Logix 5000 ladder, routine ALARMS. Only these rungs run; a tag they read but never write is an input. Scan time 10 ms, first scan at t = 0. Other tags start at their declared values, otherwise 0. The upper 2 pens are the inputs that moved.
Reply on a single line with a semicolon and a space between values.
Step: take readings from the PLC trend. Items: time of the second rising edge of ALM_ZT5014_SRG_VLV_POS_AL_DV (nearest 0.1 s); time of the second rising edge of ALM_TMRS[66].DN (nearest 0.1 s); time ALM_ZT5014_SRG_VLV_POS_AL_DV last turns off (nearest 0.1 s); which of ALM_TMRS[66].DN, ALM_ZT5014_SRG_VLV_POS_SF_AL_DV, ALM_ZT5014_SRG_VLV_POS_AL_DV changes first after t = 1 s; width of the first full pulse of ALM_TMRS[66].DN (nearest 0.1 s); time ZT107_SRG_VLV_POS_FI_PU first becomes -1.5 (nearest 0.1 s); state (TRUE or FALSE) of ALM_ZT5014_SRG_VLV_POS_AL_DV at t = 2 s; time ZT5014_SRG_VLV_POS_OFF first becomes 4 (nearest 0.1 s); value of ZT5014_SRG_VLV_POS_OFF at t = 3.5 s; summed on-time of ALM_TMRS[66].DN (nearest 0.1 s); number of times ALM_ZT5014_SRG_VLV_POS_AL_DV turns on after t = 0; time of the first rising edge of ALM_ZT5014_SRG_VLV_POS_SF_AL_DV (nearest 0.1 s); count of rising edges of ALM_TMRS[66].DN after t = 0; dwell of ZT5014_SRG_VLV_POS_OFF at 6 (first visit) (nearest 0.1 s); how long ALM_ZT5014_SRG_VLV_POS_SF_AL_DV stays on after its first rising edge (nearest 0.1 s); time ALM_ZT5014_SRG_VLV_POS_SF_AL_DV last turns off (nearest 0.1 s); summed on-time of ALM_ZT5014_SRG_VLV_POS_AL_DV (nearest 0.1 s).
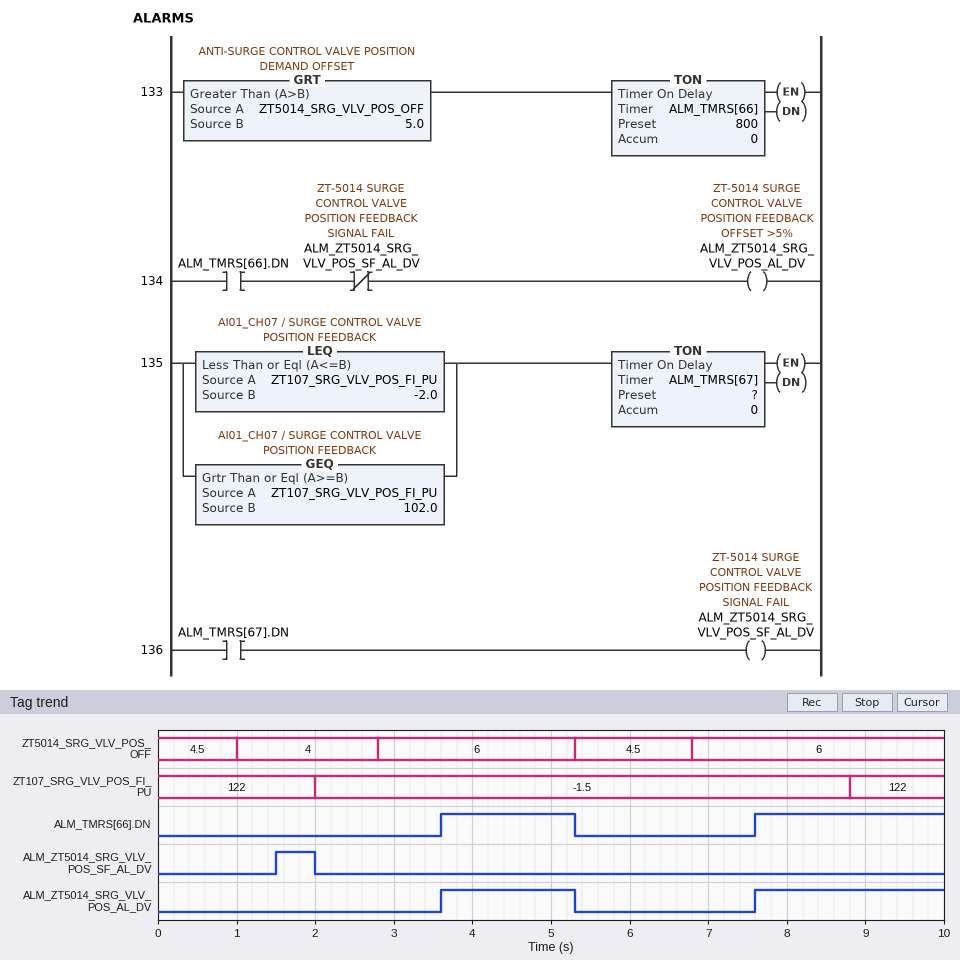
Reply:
7.6 s; 7.6 s; 5.3 s; ALM_ZT5014_SRG_VLV_POS_SF_AL_DV; 1.7 s; 2.0 s; FALSE; 1.0 s; 6; 4.1 s; 2; 1.5 s; 2; 2.5 s; 0.5 s; 2.0 s; 4.1 s
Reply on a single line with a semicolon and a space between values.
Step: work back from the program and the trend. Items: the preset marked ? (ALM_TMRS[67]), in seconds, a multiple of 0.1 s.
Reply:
1.5 s
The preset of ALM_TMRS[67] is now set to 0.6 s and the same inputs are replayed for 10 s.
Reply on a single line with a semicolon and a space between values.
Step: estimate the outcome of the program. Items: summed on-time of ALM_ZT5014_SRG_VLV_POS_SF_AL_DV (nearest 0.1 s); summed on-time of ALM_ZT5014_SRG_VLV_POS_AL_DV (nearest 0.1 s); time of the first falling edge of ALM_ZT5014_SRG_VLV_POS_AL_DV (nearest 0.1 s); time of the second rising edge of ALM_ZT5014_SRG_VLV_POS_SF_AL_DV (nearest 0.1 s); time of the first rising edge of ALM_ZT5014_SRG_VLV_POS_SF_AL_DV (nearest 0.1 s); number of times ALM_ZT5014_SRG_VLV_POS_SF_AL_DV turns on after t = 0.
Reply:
2.0 s; 3.5 s; 5.3 s; 9.4 s; 0.6 s; 2
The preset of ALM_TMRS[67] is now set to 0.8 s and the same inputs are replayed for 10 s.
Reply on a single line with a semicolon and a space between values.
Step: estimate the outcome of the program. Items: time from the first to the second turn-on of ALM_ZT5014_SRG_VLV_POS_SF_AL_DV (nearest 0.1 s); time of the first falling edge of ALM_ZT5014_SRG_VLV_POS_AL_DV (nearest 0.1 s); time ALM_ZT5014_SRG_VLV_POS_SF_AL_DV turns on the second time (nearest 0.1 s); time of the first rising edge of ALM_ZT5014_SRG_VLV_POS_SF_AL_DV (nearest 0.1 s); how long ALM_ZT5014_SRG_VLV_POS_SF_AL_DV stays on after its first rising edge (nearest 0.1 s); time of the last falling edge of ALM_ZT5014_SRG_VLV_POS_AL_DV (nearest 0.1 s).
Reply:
8.8 s; 5.3 s; 9.6 s; 0.8 s; 1.2 s; 9.6 s
